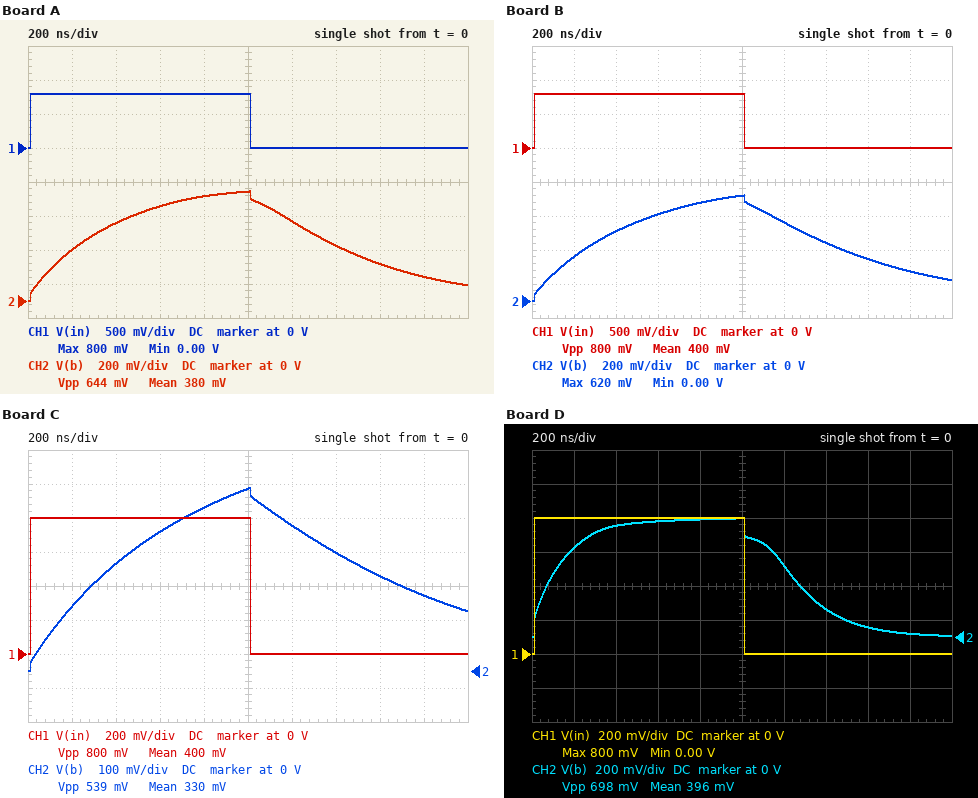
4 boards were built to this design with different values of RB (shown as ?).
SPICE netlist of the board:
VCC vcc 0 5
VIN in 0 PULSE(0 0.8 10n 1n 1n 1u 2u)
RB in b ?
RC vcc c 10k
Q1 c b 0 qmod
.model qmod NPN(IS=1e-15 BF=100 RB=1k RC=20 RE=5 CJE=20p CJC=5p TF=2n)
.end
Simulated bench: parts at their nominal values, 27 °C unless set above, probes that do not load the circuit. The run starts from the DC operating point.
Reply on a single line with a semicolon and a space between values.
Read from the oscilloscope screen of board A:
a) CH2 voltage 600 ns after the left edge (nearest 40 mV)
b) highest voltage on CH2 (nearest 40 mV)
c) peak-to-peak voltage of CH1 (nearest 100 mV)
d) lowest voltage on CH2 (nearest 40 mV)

560 mV; 640 mV; 800 mV; 0 V
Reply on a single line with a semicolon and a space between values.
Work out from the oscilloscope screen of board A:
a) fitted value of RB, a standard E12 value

18 kΩ
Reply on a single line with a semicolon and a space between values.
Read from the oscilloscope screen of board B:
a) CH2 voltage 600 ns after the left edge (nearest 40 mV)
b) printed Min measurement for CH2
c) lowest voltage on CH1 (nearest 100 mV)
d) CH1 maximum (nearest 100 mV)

520 mV; 0.00 V; 0 V; 800 mV
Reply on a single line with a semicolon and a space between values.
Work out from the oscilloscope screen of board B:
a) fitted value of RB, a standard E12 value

22 kΩ
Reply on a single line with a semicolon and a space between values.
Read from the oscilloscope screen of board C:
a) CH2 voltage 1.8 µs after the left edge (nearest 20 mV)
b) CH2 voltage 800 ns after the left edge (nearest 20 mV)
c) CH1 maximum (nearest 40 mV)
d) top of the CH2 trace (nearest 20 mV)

220 mV; 480 mV; 800 mV; 540 mV
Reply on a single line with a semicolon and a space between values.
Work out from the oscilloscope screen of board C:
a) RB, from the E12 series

33 kΩ
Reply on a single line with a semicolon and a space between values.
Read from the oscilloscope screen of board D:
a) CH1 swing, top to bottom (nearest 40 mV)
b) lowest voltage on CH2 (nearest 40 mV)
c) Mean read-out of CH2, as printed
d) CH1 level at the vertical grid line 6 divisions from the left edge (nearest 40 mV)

800 mV; 0 V; 396 mV; 0 V
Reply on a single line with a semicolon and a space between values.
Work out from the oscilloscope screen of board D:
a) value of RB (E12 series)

6.8 kΩ
